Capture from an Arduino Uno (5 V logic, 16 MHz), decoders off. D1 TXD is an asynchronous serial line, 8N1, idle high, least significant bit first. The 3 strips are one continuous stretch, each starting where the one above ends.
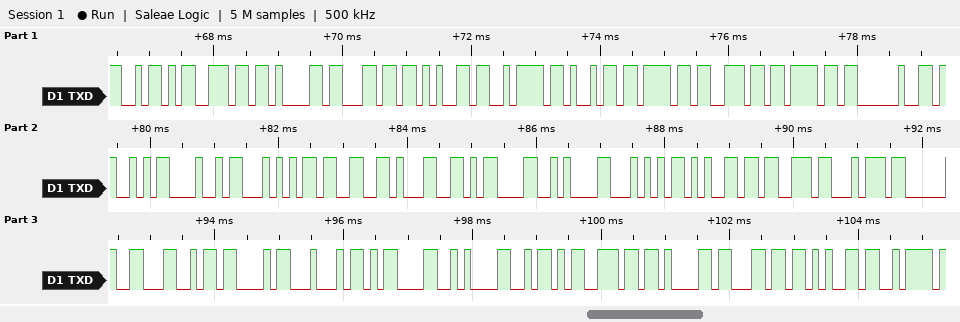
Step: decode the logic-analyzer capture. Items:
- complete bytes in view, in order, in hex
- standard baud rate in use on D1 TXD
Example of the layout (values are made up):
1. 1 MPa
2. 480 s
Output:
1. 5A 6E 61 6C 65 7A 69 6F 6E 6F 20 53 48 54 33 31 0D 0A 54 65 73 74 20 4C 43 44 0D 0A 5A 6E 61 6C 65 7A
2. 9600 baud
